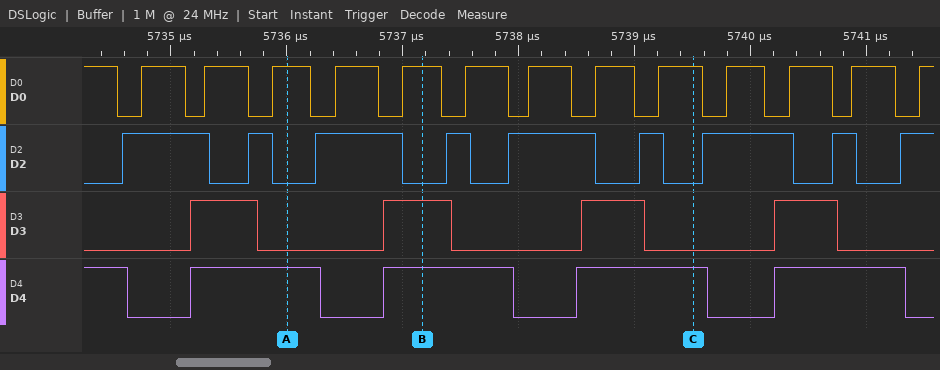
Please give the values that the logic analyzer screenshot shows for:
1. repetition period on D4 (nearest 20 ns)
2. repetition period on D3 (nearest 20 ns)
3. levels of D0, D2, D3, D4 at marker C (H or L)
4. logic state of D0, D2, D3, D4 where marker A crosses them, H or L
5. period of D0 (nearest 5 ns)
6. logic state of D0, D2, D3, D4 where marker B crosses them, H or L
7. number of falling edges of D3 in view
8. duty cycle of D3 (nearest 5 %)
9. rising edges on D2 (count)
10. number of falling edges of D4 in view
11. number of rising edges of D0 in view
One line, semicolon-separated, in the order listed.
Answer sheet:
1680 ns; 1680 ns; D0=H, D2=L, D3=L, D4=H; D0=H, D2=L, D3=L, D4=H; 560 ns; D0=H, D2=L, D3=H, D4=H; 4; 35 %; 9; 5; 13
